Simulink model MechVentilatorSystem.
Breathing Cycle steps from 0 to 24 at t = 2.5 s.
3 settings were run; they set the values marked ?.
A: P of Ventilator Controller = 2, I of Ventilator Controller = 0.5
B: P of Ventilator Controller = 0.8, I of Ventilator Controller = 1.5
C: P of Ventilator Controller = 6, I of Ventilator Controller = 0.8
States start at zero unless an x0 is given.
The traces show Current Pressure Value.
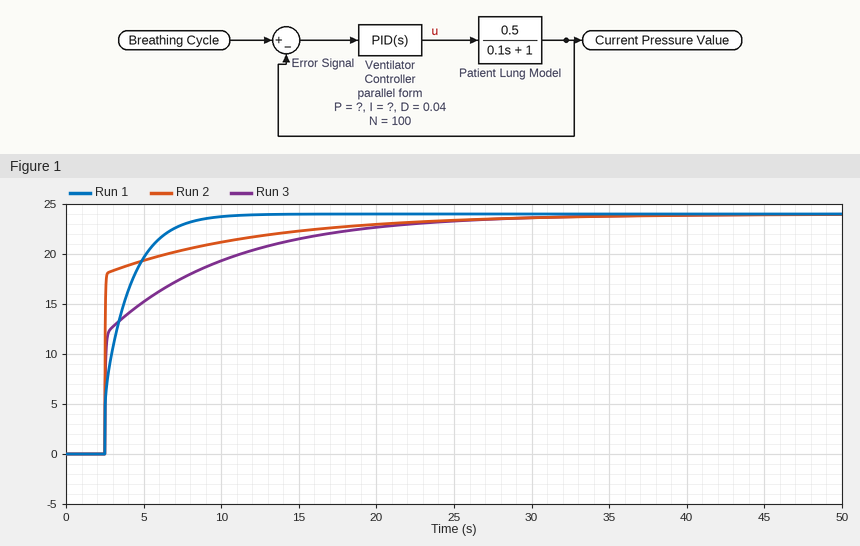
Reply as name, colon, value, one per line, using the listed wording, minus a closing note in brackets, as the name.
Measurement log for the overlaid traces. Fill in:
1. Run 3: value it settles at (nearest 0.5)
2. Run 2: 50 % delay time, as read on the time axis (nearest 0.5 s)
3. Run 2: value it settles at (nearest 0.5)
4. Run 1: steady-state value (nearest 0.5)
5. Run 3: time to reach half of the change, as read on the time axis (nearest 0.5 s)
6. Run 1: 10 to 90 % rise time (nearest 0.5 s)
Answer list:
Run 3: value it settles at: 24.0
Run 2: 50 % delay time, as read on the time axis: 2.5 s
Run 2: value it settles at: 24.0
Run 1: steady-state value: 24.0
Run 3: time to reach half of the change, as read on the time axis: 2.5 s
Run 1: 10 to 90 % rise time: 3.5 s
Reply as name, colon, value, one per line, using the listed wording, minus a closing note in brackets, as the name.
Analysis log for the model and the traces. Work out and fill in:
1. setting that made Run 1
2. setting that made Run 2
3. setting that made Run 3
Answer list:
setting that made Run 1: B
setting that made Run 2: C
setting that made Run 3: A
